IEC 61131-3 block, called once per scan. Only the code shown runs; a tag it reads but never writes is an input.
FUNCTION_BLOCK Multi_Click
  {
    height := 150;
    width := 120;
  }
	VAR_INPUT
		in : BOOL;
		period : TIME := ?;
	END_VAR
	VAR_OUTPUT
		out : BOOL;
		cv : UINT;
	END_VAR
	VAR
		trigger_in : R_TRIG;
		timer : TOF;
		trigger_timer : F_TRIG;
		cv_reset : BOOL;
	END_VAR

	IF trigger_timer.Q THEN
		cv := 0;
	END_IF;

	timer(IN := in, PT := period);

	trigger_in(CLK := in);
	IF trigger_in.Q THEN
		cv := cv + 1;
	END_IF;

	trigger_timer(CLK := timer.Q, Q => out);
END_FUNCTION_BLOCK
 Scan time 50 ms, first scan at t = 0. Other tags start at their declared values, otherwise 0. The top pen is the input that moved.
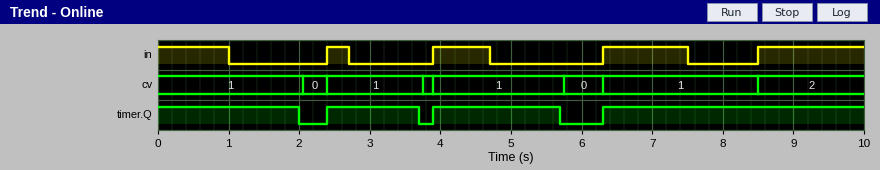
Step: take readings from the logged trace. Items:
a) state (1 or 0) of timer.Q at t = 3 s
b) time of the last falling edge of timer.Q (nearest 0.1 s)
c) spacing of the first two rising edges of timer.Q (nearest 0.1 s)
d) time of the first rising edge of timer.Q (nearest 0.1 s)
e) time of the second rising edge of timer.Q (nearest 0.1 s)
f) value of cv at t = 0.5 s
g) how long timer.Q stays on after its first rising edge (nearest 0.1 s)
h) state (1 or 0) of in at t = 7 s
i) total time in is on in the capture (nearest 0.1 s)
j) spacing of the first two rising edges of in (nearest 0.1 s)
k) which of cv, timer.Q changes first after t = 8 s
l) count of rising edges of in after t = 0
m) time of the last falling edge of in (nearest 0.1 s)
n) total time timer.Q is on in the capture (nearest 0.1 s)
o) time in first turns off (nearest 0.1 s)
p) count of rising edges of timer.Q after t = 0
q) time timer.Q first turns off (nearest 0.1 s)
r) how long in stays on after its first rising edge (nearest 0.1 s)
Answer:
1
5.7 s
1.5 s
2.4 s
3.9 s
1
1.3 s
1
4.8 s
1.5 s
cv
4
7.5 s
8.8 s
1.0 s
3
2.0 s
0.3 s
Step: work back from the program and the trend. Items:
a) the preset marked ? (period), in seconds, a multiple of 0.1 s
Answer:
1.0 s
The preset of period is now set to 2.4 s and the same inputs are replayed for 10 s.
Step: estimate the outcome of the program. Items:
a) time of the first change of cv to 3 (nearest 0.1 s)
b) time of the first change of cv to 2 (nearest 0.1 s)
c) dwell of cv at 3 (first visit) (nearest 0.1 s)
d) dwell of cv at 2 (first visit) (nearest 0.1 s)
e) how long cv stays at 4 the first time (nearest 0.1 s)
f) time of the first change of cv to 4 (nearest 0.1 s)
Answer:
3.9 s
2.4 s
2.4 s
1.5 s
2.2 s
6.3 s
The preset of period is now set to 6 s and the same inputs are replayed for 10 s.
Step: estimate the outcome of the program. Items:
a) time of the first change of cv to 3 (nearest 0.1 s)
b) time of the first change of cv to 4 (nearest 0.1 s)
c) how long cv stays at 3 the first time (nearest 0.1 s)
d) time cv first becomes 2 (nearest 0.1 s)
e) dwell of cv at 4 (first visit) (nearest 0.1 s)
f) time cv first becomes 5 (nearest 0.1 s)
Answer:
3.9 s
6.3 s
2.4 s
2.4 s
2.2 s
8.5 s
